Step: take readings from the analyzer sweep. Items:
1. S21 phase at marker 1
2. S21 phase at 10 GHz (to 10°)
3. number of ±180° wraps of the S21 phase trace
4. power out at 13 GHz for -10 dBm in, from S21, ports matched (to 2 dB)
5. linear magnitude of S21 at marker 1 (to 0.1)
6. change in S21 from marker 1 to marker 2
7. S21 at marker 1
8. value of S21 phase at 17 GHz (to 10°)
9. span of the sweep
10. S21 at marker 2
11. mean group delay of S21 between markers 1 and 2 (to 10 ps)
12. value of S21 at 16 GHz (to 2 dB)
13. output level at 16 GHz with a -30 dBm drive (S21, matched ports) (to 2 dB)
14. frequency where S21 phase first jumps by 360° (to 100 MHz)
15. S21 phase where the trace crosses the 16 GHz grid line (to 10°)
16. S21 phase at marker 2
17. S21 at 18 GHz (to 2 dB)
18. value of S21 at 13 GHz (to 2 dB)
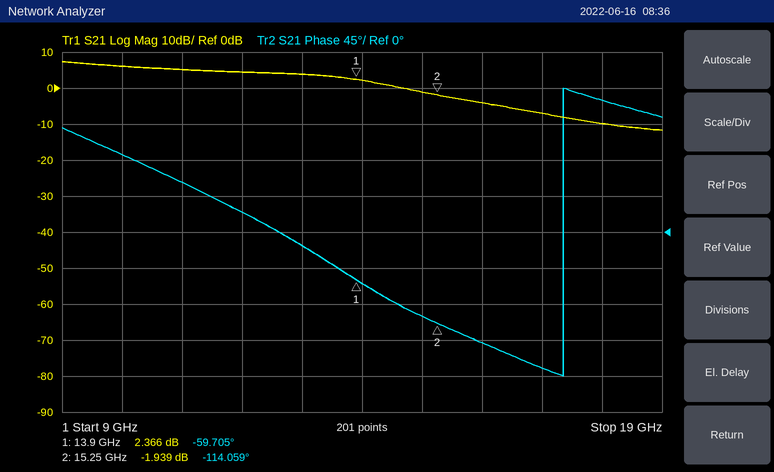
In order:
-59.705°
100°
1
-6 dBm
1.3
-4.305 dB
2.366 dB
-170°
10 GHz
-1.939 dB
110 ps
-4 dB
-34 dBm
17.4 GHz
-140°
-114.059°
-10 dB
4 dB
